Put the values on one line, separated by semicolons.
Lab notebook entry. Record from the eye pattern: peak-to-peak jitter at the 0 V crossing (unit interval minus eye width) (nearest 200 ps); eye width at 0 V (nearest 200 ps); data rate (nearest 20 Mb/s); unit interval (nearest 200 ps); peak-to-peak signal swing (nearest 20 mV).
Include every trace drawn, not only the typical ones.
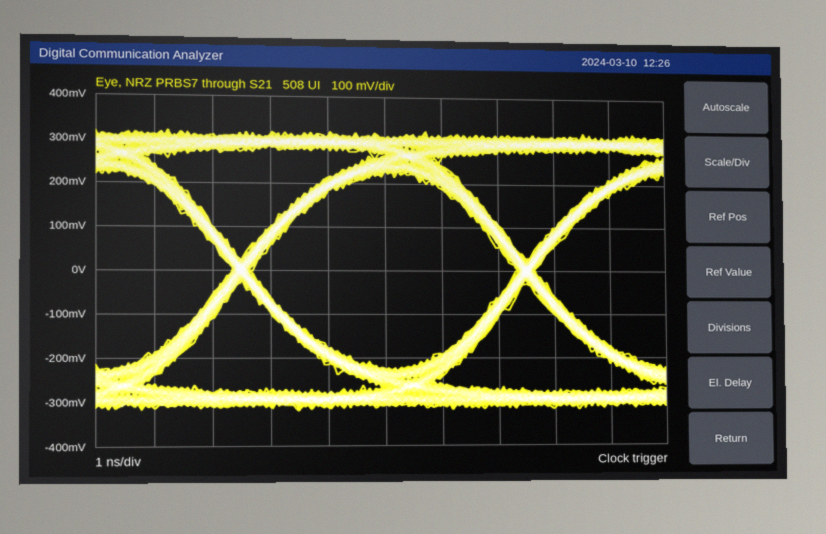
400 ps; 4.6 ns; 200 Mb/s; 5.0 ns; 640 mV
